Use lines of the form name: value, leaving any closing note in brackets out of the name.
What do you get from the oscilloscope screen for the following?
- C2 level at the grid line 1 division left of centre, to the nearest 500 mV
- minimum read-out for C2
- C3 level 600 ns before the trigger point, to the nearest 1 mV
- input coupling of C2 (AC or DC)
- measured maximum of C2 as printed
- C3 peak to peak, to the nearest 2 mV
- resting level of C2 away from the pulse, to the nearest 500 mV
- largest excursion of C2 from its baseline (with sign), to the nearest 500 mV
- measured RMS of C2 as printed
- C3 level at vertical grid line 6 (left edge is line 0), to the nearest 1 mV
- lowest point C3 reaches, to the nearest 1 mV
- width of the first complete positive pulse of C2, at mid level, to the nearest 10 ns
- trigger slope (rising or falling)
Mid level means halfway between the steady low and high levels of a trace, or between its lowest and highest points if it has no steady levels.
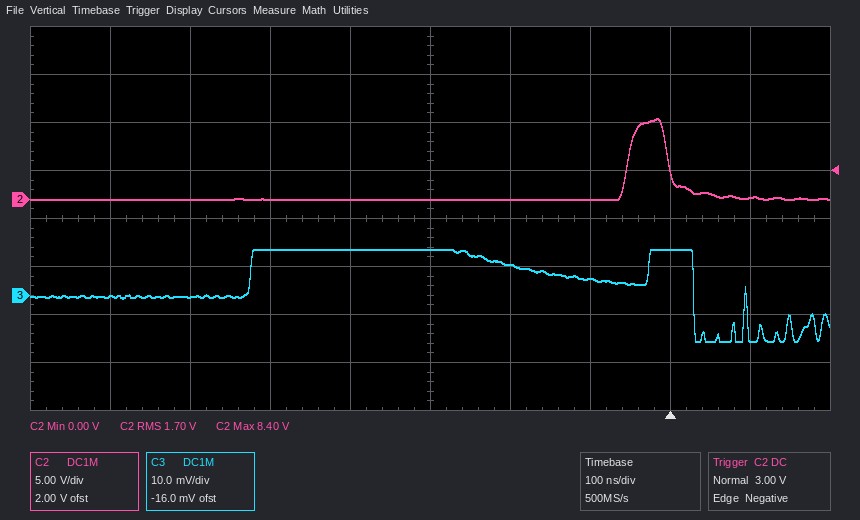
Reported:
C2 level at the grid line 1 division left of centre, to the nearest 500 mV: 0.0 V
minimum read-out for C2: 0.00 V
C3 level 600 ns before the trigger point, to the nearest 1 mV: 0 mV
input coupling of C2: DC
measured maximum of C2 as printed: 8.40 V
C3 peak to peak, to the nearest 2 mV: 20 mV
resting level of C2 away from the pulse, to the nearest 500 mV: 0.0 V
largest excursion of C2 from its baseline (with sign), to the nearest 500 mV: +8.5 V
measured RMS of C2 as printed: 1.70 V
C3 level at vertical grid line 6 (left edge is line 0), to the nearest 1 mV: 6 mV
lowest point C3 reaches, to the nearest 1 mV: -10 mV
width of the first complete positive pulse of C2, at mid level, to the nearest 10 ns: 50 ns
trigger slope: falling
